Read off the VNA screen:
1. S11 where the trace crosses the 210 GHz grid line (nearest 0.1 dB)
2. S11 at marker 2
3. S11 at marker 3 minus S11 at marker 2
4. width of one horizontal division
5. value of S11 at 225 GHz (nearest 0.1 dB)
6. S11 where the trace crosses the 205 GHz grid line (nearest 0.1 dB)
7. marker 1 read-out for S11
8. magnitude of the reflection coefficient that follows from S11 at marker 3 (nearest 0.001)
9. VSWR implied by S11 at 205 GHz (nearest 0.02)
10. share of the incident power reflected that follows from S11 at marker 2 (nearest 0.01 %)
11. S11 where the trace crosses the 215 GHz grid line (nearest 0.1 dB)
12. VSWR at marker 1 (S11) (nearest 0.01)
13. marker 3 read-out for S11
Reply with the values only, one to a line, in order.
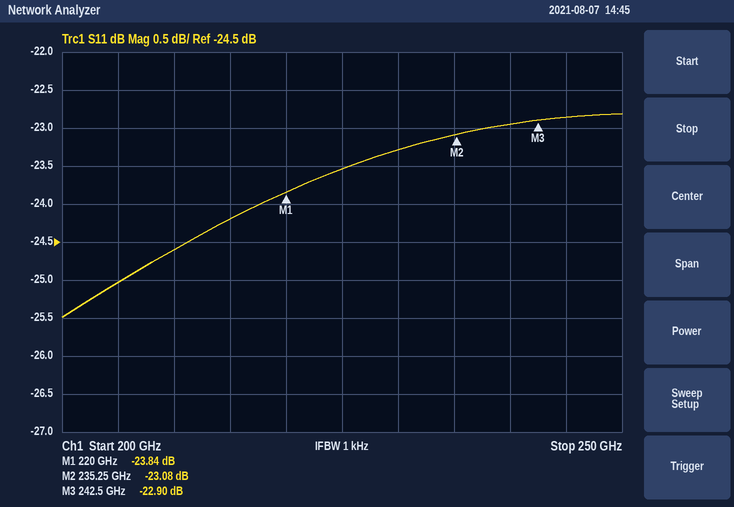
-24.6 dB
-23.08 dB
0.18 dB
5 GHz
-23.5 dB
-25.0 dB
-23.84 dB
0.072
1.12
0.49 %
-24.2 dB
1.14
-22.90 dB
